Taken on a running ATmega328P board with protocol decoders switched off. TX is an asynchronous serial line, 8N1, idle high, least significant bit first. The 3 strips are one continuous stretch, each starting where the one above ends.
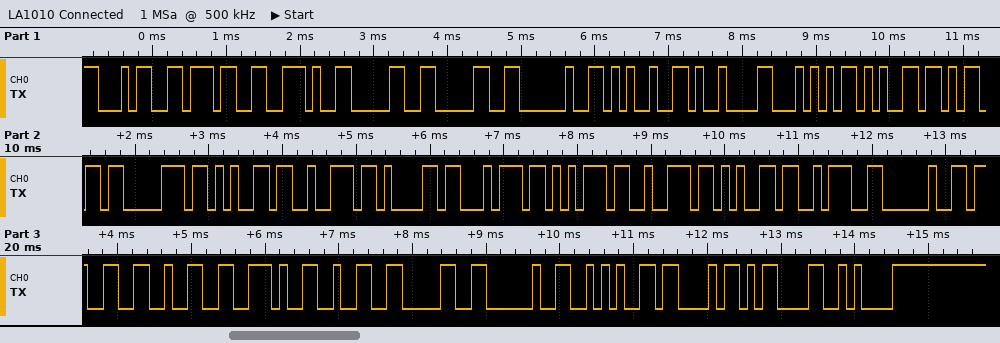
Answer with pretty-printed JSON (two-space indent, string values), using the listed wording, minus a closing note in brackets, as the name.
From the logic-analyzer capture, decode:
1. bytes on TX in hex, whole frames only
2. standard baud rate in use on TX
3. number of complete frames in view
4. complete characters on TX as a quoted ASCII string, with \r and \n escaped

{
  "bytes on TX in hex, whole frames only": "0x34 0x37 0x2E 0x30 0x30 0x20 0x25 0x09 0x54 0x65 0x6D 0x70 0x65 0x72 0x61 0x74 0x75 0x72 0x65 0x3A 0x20 0x33 0x32 0x2E 0x32 0x30 0x20 0x2A 0x43 0x0D 0x0A",
  "standard baud rate in use on TX": "9600 baud",
  "number of complete frames in view": "31",
  "complete characters on TX as a quoted ASCII string, with \\r and \\n escaped": "\"47.00 %\\tTemperature: 32.20 *C\\r\\n\""
}
